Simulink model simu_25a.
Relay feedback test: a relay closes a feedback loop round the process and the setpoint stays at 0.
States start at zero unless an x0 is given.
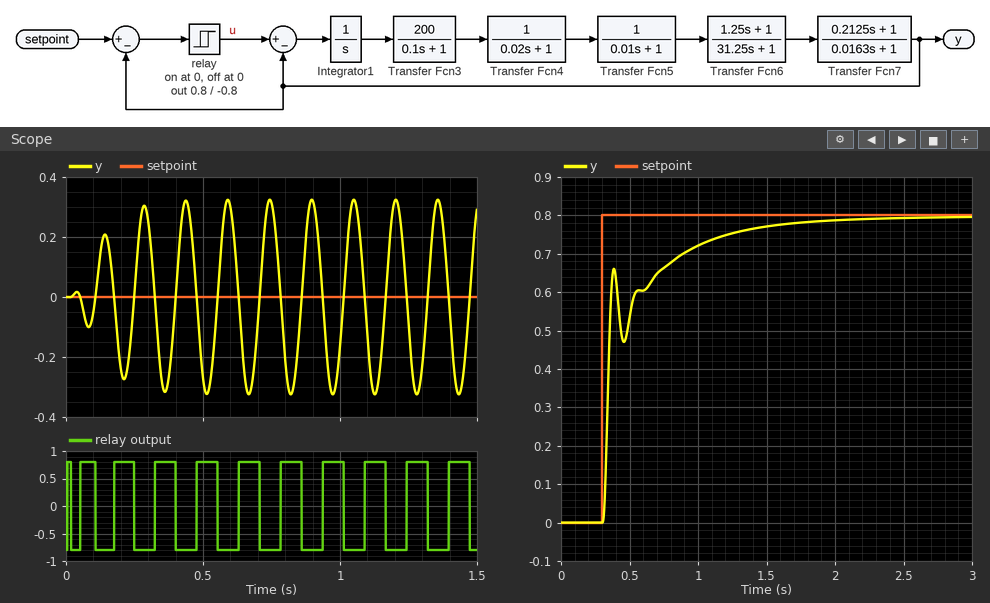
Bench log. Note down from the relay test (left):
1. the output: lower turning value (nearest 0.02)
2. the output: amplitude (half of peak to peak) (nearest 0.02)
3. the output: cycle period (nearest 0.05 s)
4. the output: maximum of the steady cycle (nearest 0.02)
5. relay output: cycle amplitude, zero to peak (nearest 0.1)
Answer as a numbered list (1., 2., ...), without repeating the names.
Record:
1. -0.32
2. 0.32
3. 0.15 s
4. 0.32
5. 0.8
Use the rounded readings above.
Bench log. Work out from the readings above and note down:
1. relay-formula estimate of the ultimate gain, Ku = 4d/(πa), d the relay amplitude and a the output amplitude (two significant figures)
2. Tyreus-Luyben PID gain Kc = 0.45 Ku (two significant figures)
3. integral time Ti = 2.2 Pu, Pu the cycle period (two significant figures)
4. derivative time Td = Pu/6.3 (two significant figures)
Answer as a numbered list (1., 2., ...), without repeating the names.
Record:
1. 3.2
2. 1.4
3. 0.33 s
4. 0.024 s
